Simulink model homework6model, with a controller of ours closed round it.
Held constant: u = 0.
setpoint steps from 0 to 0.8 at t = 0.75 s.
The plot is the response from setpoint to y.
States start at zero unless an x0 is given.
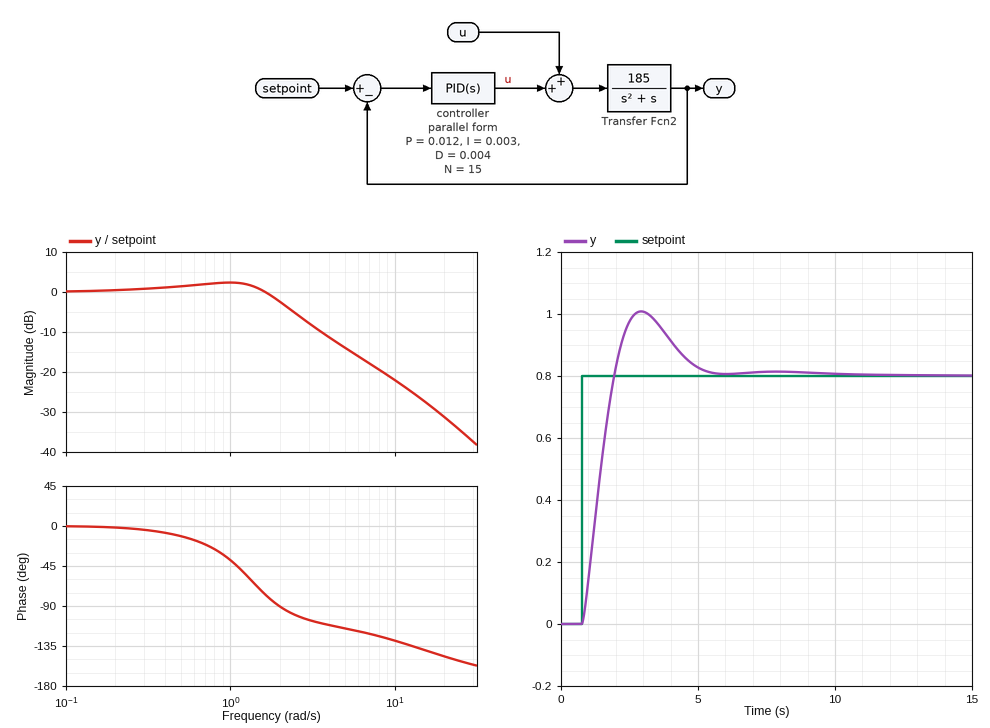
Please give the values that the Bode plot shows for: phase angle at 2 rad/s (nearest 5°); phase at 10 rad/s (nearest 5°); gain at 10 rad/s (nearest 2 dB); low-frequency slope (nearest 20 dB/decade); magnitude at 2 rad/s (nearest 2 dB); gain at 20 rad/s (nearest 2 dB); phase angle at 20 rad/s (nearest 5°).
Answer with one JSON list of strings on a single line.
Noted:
["-90°", "-130°", "-22 dB", "0 dB/decade", "-2 dB", "-32 dB", "-145°"]
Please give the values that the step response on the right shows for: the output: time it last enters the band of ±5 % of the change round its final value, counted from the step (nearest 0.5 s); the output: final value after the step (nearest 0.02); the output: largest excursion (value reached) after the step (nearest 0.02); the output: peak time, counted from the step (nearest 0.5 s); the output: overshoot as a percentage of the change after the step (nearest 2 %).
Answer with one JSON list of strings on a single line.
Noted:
["4.0 s", "0.80", "1.00", "2.0 s", "26 %"]
